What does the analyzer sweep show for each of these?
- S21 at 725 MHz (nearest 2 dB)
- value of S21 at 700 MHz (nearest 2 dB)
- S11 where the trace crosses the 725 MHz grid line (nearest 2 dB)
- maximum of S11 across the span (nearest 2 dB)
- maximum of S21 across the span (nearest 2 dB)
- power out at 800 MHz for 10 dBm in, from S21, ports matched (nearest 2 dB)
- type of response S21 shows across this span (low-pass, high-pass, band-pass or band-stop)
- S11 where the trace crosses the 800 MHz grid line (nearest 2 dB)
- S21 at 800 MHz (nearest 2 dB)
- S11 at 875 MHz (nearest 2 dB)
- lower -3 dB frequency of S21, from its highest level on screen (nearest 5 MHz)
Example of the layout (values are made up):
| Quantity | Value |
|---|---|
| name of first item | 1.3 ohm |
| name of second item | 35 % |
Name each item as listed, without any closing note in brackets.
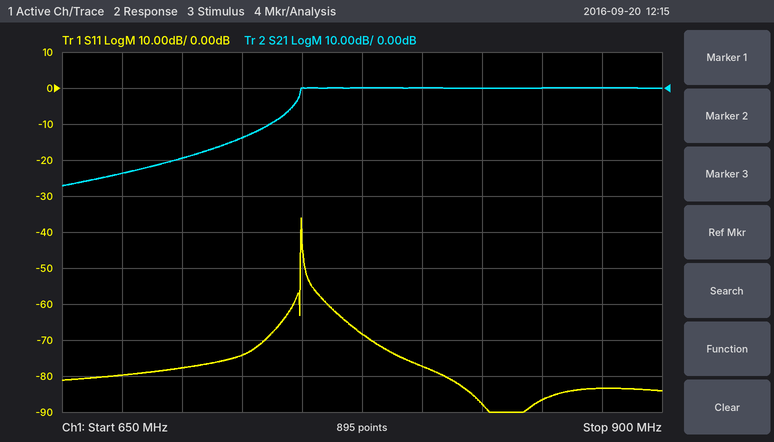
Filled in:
| Quantity | Value |
|---|---|
| S21 at 725 MHz | -14 dB |
| value of S21 at 700 MHz | -20 dB |
| S11 where the trace crosses the 725 MHz grid line | -74 dB |
| maximum of S11 across the span | -36 dB |
| maximum of S21 across the span | 0 dB |
| power out at 800 MHz for 10 dBm in, from S21, ports matched | 10 dBm |
| type of response S21 shows across this span | high-pass |
| S11 where the trace crosses the 800 MHz grid line | -78 dB |
| S21 at 800 MHz | 0 dB |
| S11 at 875 MHz | -84 dB |
| lower -3 dB frequency of S21, from its highest level on screen | 750 MHz |
